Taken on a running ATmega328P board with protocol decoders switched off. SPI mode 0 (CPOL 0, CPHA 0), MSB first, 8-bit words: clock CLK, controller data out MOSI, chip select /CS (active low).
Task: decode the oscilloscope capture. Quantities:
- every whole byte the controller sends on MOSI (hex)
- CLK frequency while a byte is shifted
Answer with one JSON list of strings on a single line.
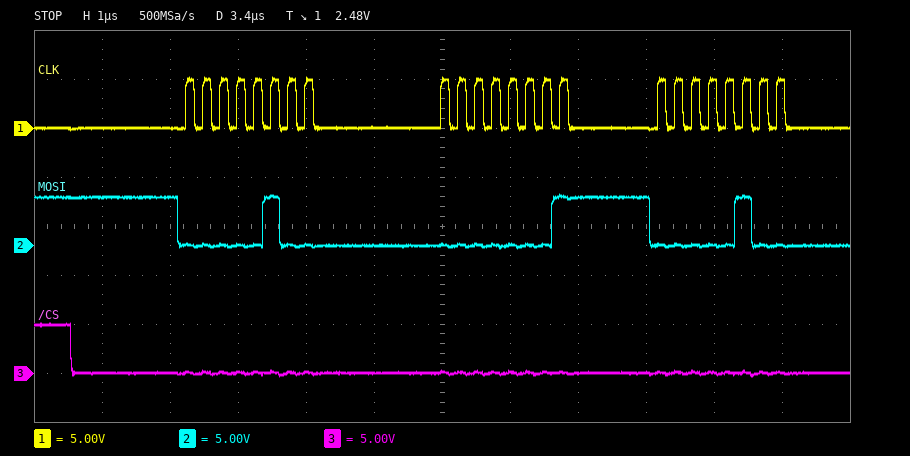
["0x04 0x01 0x04", "4 MHz"]
